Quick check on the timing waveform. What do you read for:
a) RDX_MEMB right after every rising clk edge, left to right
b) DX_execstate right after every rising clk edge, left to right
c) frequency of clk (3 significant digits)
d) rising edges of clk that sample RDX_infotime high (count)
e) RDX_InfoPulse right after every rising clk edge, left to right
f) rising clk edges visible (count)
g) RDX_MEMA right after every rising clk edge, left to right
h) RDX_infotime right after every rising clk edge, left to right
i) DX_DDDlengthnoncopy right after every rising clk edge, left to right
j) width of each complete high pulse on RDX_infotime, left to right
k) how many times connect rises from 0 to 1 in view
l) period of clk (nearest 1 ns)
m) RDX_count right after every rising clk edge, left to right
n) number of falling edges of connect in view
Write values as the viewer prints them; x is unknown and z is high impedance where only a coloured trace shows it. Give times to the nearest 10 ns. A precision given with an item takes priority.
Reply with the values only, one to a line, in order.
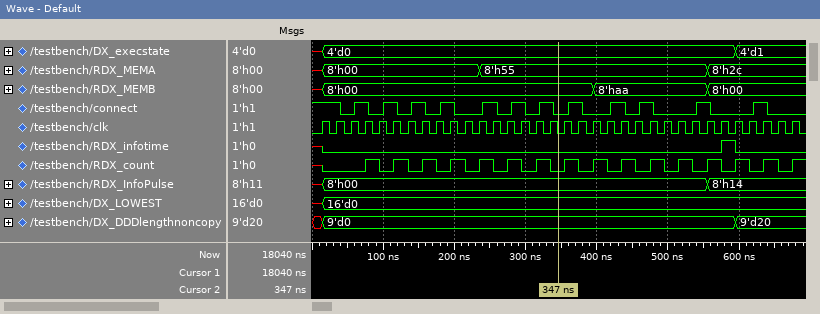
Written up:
8'h00, 8'h00, 8'h00, 8'h00, 8'h00, 8'h00, 8'h00, 8'h00, 8'h00, 8'h00, 8'h00, 8'h00, 8'h00, 8'h00, 8'h00, 8'h00, 8'h00, 8'h00, 8'h00, 8'haa, 8'haa, 8'haa, 8'haa, 8'haa, 8'haa, 8'haa, 8'haa, 8'h00, 8'h00, 8'h00, 8'h00, 8'h00, 8'h00, 8'h00
4'd0, 4'd0, 4'd0, 4'd0, 4'd0, 4'd0, 4'd0, 4'd0, 4'd0, 4'd0, 4'd0, 4'd0, 4'd0, 4'd0, 4'd0, 4'd0, 4'd0, 4'd0, 4'd0, 4'd0, 4'd0, 4'd0, 4'd0, 4'd0, 4'd0, 4'd0, 4'd0, 4'd0, 4'd0, 4'd1, 4'd1, 4'd1, 4'd1, 4'd1
50.0 MHz
1
8'h00, 8'h00, 8'h00, 8'h00, 8'h00, 8'h00, 8'h00, 8'h00, 8'h00, 8'h00, 8'h00, 8'h00, 8'h00, 8'h00, 8'h00, 8'h00, 8'h00, 8'h00, 8'h00, 8'h00, 8'h00, 8'h00, 8'h00, 8'h00, 8'h00, 8'h00, 8'h00, 8'h14, 8'h14, 8'h14, 8'h14, 8'h14, 8'h14, 8'h14
34
8'h00, 8'h00, 8'h00, 8'h00, 8'h00, 8'h00, 8'h00, 8'h00, 8'h00, 8'h00, 8'h00, 8'h55, 8'h55, 8'h55, 8'h55, 8'h55, 8'h55, 8'h55, 8'h55, 8'h55, 8'h55, 8'h55, 8'h55, 8'h55, 8'h55, 8'h55, 8'h55, 8'h2c, 8'h2c, 8'h2c, 8'h2c, 8'h2c, 8'h2c, 8'h2c
0 0 0 0 0 0 0 0 0 0 0 0 0 0 0 0 0 0 0 0 0 0 0 0 0 0 0 0 1 0 0 0 0 0
9'd0, 9'd0, 9'd0, 9'd0, 9'd0, 9'd0, 9'd0, 9'd0, 9'd0, 9'd0, 9'd0, 9'd0, 9'd0, 9'd0, 9'd0, 9'd0, 9'd0, 9'd0, 9'd0, 9'd0, 9'd0, 9'd0, 9'd0, 9'd0, 9'd0, 9'd0, 9'd0, 9'd0, 9'd0, 9'd20, 9'd20, 9'd20, 9'd20, 9'd20
20 ns
12
20 ns
0 0 0 1 0 1 0 1 0 1 0 1 0 1 0 1 0 1 0 1 0 1 0 1 0 1 0 1 0 1 0 1 0 1
13
